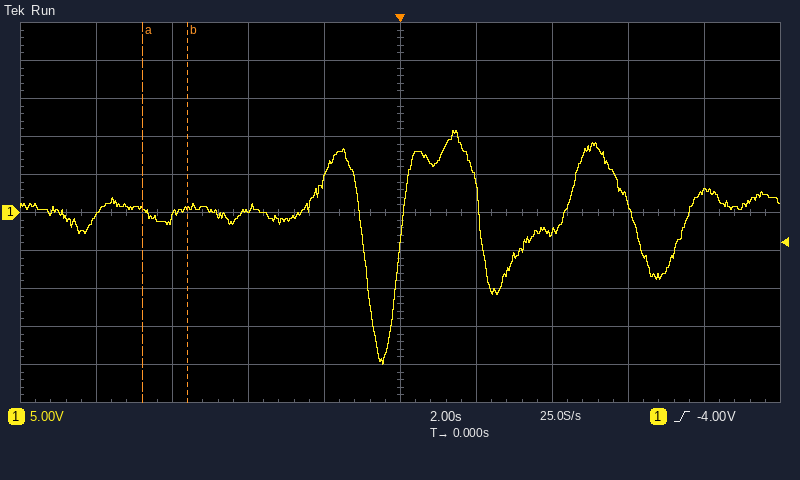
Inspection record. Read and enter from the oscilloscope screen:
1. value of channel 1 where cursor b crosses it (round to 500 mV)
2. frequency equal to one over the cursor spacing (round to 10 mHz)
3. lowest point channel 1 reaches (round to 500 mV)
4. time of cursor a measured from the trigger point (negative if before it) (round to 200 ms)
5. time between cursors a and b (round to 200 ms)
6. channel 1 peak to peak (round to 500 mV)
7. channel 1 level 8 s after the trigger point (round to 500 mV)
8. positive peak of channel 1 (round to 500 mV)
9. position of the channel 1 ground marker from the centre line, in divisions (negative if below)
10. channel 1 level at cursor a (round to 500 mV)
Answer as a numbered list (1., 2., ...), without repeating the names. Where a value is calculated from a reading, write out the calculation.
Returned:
1. 500 mV
2. 1 / 1.2 s ≈ 830 mHz
3. -20.0 V
4. -6.8 s
5. 1.2 s
6. 11.0 V − (-20.0 V) = 31.0 V
7. 3.0 V
8. 11.0 V
9. 0.0 div
10. 500 mV
